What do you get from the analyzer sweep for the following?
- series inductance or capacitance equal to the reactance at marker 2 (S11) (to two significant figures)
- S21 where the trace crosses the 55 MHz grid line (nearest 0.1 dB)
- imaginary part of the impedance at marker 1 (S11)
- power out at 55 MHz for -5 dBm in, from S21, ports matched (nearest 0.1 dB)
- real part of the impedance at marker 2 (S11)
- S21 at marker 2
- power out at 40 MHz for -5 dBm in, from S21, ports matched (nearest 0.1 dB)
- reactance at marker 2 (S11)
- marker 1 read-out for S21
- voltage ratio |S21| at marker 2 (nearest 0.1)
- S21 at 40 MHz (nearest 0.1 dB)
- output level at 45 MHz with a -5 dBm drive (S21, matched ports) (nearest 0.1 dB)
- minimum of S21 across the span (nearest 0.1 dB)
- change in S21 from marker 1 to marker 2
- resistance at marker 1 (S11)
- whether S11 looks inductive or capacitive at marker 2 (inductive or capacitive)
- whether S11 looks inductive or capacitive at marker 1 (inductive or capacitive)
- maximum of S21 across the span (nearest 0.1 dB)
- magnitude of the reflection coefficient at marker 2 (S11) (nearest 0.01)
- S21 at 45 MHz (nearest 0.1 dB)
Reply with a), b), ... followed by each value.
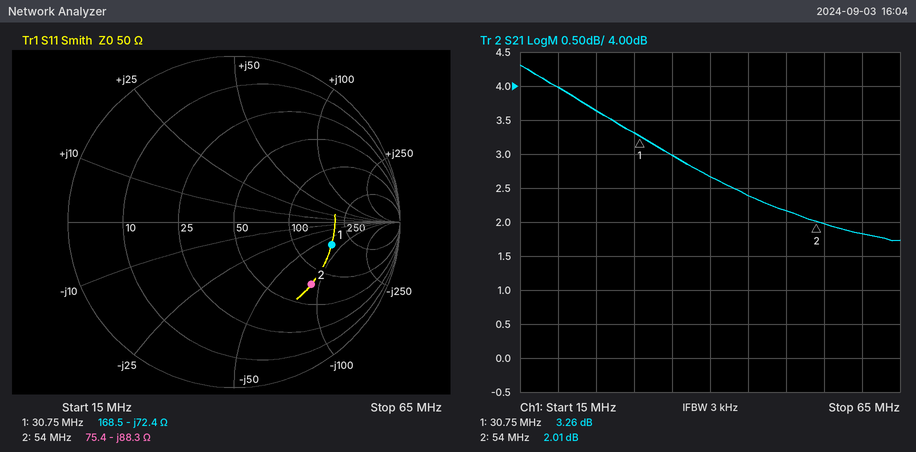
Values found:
a) 33 pF
b) 2.0 dB
c) -72.4 Ω
d) -3.0 dBm
e) 75.4 Ω
f) 2.01 dB
g) -2.3 dBm
h) -88.3 Ω
i) 3.26 dB
j) 1.3
k) 2.7 dB
l) -2.6 dBm
m) 1.7 dB
n) -1.25 dB
o) 168.5 Ω
p) capacitive
q) capacitive
r) 4.3 dB
s) 0.60
t) 2.4 dB
